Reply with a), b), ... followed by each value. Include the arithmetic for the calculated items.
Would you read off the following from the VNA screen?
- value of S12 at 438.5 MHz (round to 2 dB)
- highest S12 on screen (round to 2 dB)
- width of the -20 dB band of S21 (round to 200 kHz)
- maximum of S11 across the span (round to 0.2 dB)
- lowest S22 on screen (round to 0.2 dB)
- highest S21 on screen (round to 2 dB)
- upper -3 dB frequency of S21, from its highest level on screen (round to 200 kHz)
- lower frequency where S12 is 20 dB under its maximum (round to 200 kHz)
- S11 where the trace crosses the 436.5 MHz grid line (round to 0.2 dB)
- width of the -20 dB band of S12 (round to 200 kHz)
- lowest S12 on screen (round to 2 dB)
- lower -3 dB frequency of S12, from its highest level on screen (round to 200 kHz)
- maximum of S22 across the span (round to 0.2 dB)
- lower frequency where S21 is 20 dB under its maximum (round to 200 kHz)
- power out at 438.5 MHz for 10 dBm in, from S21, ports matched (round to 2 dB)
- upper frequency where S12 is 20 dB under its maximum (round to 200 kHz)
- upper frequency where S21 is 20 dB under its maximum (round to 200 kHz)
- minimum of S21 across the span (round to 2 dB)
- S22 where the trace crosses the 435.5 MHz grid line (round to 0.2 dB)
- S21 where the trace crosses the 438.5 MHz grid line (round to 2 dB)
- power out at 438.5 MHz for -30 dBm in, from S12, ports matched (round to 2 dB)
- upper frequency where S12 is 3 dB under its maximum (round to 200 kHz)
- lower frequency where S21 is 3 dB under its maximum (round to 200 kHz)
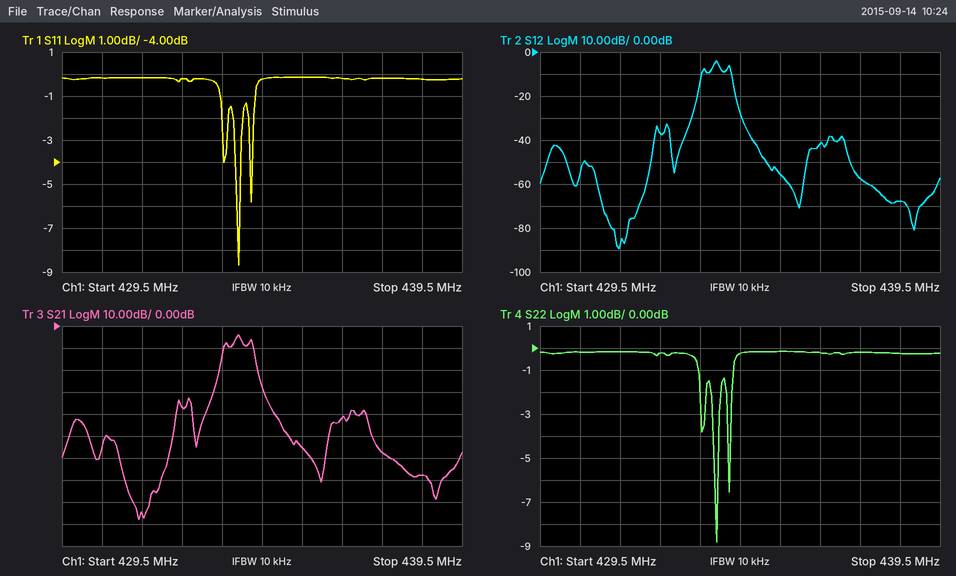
a) -68 dB
b) -4 dB
c) 434.4 MHz − 433.4 MHz = 1.0 MHz
d) -0.2 dB
e) -8.8 dB
f) -4 dB
g) 434.0 MHz
h) 433.4 MHz
i) -0.2 dB
j) 434.4 MHz − 433.4 MHz = 1.0 MHz
k) -90 dB
l) 433.8 MHz
m) -0.2 dB
n) 433.4 MHz
o) 10 dBm + (-68 dB) = -58 dBm
p) 434.4 MHz
q) 434.4 MHz
r) -88 dB
s) -0.2 dB
t) -68 dB
u) -30 dBm + (-68 dB) = -98 dBm
v) 434.0 MHz
w) 433.8 MHz
